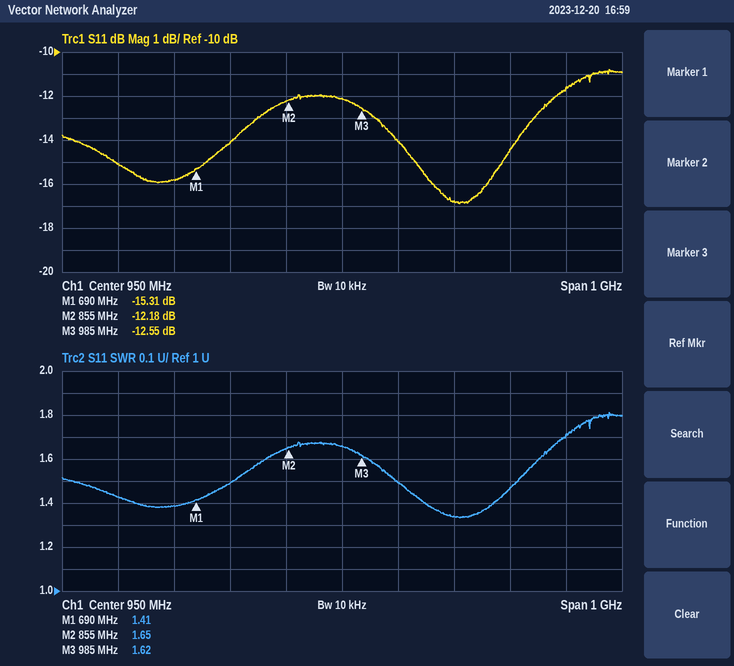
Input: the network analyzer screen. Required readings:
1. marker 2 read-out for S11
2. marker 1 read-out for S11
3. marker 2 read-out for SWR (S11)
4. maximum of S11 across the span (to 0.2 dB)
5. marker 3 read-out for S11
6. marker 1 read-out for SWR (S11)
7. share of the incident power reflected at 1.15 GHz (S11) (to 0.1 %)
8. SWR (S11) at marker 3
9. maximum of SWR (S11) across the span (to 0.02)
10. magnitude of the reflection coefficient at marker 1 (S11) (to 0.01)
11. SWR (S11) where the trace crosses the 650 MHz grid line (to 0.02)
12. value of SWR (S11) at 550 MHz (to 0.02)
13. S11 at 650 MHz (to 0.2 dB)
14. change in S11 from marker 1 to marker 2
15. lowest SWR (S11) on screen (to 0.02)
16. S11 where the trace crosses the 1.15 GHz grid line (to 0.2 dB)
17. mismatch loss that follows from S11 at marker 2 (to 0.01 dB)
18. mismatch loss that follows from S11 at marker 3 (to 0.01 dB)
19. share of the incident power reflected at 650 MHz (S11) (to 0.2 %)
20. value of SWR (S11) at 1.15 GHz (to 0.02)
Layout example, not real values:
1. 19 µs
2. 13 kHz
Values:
1. -12.18 dB
2. -15.31 dB
3. 1.65
4. -10.8 dB
5. -12.55 dB
6. 1.41
7. 2.1 %
8. 1.62
9. 1.82
10. 0.17
11. 1.38
12. 1.42
13. -15.8 dB
14. 3.13 dB
15. 1.34
16. -16.8 dB
17. 0.27 dB
18. 0.25 dB
19. 2.6 %
20. 1.34
